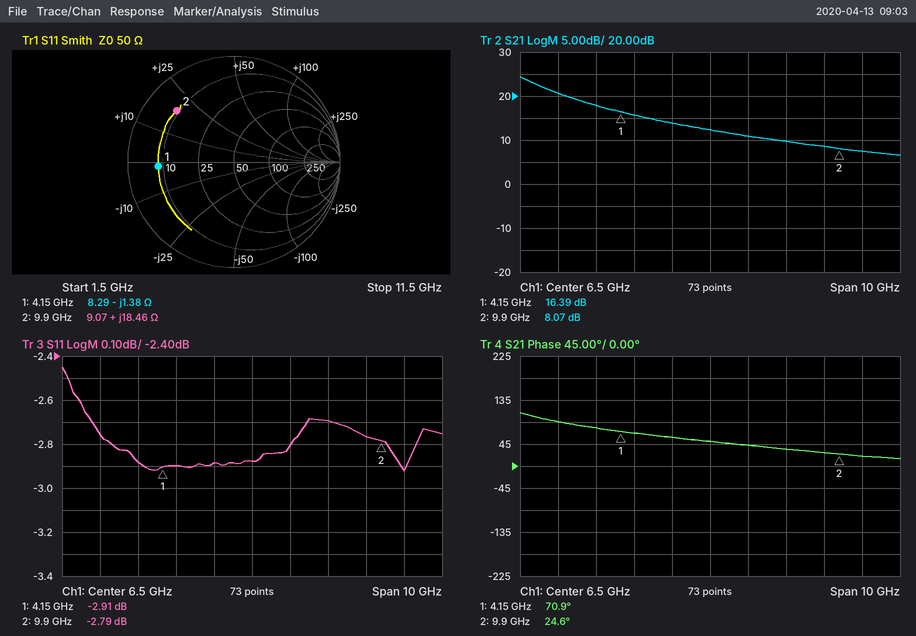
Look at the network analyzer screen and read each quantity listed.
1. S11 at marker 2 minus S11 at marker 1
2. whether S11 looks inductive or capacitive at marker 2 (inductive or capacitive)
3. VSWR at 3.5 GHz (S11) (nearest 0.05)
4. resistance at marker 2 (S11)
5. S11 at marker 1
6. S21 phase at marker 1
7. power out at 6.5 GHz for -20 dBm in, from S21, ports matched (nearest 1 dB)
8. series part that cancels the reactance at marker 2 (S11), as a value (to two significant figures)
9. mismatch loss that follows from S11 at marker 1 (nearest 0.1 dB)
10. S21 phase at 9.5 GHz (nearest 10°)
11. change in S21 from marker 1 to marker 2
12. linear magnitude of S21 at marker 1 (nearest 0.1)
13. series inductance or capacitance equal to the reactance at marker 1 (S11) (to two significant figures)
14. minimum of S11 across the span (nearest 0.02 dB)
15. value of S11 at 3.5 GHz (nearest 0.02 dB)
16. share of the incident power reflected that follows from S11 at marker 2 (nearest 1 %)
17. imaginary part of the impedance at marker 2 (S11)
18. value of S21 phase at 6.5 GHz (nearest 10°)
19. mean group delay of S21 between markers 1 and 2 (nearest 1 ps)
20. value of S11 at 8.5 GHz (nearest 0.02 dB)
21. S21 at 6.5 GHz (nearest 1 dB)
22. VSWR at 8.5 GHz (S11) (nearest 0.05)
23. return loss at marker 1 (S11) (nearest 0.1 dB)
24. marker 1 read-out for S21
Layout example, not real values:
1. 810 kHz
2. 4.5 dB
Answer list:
1. 0.12 dB
2. inductive
3. 6.10
4. 9.07 Ω
5. -2.91 dB
6. 70.9°
7. -8 dBm
8. 870 fF
9. 3.1 dB
10. 30°
11. -8.32 dB
12. 6.6
13. 28 pF
14. -2.92 dB
15. -2.88 dB
16. 53 %
17. +18.46 Ω
18. 50°
19. 22 ps
20. -2.70 dB
21. 12 dB
22. 6.50
23. 2.9 dB
24. 16.39 dB
